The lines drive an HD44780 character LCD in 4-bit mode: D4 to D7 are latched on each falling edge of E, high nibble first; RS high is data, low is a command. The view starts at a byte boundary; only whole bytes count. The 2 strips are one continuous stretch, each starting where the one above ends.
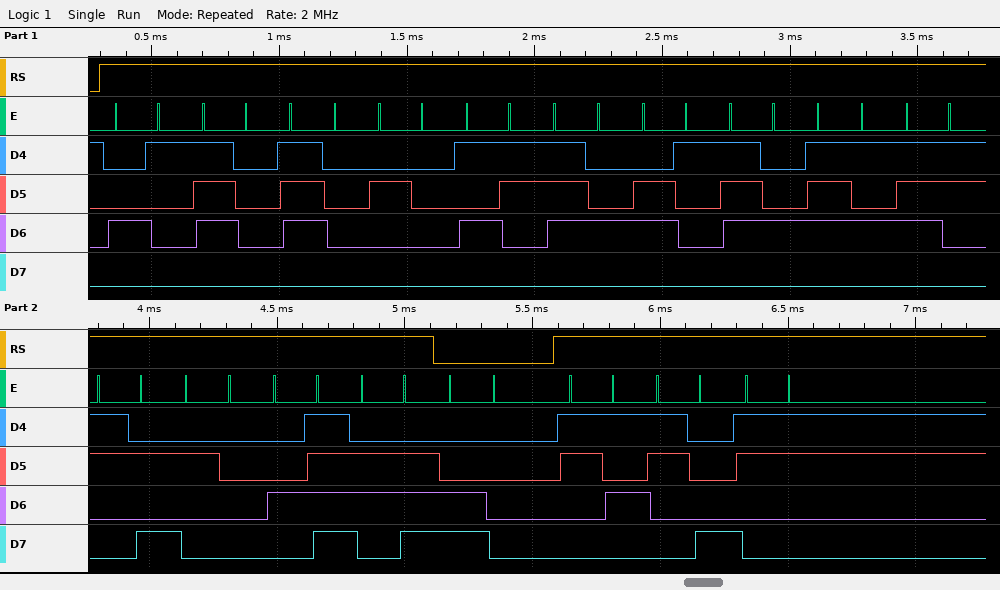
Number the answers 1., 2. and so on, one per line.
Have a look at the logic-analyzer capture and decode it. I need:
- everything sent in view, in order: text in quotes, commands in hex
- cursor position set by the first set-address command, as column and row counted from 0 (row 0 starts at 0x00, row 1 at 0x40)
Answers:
1. "App Status: On" 0xC0 "583"
2. column 0, row 1
